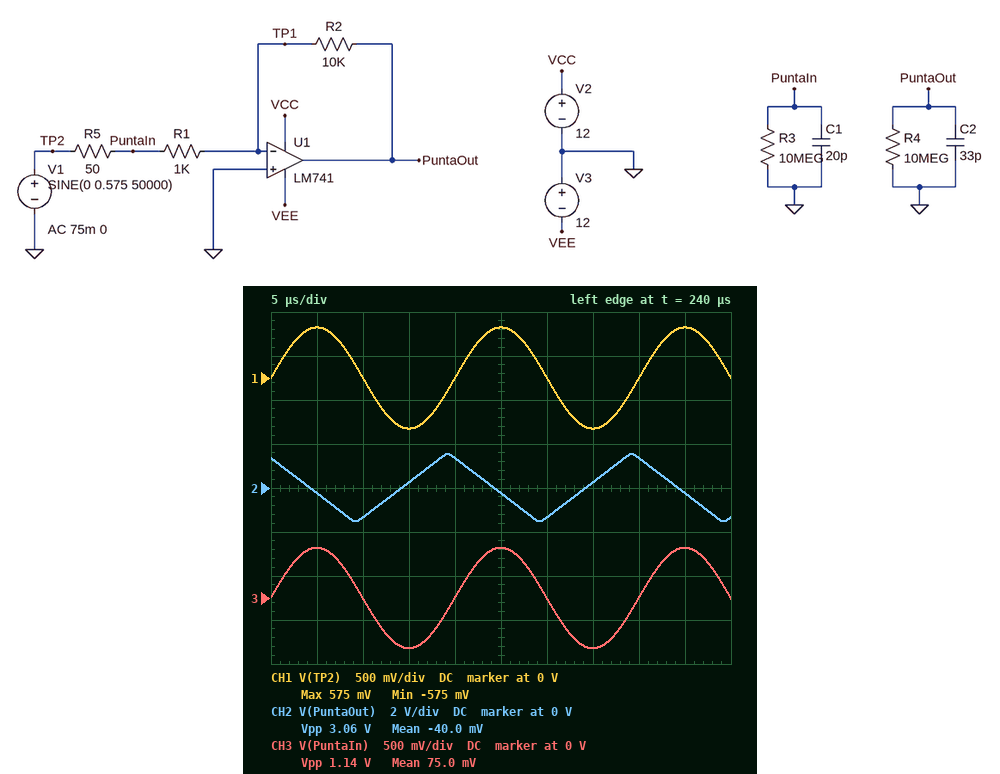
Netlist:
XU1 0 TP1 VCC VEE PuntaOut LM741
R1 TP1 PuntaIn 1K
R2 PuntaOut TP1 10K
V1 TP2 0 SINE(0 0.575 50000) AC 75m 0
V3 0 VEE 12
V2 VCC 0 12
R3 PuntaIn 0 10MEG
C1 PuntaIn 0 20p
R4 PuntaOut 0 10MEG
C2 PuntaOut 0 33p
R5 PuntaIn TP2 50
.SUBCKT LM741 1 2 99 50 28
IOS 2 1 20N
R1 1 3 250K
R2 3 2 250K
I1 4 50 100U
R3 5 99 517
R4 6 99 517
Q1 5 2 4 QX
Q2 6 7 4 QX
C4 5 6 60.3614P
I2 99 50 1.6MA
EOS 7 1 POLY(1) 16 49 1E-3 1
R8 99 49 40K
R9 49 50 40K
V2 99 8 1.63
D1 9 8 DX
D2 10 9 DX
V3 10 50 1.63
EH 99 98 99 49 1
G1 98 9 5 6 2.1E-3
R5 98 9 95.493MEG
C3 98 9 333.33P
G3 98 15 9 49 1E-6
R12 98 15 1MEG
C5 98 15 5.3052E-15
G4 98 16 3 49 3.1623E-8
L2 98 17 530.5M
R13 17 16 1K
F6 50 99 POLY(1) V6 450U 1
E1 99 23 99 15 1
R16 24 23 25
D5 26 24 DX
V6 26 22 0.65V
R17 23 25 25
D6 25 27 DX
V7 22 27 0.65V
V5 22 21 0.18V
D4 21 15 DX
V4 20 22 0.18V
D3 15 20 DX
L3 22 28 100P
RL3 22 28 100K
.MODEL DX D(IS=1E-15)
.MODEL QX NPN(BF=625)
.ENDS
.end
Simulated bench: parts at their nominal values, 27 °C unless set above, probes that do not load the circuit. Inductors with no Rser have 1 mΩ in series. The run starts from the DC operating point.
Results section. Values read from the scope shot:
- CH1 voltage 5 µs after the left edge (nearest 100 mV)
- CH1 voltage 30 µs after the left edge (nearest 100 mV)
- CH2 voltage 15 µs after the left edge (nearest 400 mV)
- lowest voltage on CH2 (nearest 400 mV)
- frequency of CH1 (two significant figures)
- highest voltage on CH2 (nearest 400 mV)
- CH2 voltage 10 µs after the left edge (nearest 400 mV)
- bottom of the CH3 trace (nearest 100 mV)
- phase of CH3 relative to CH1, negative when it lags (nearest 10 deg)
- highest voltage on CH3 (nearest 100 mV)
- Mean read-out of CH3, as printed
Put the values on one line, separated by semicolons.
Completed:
600 mV; 0 V; 400 mV; -1.6 V; 50 kHz; 1.6 V; -1.2 V; -600 mV; 0 deg; 600 mV; 75.0 mV
